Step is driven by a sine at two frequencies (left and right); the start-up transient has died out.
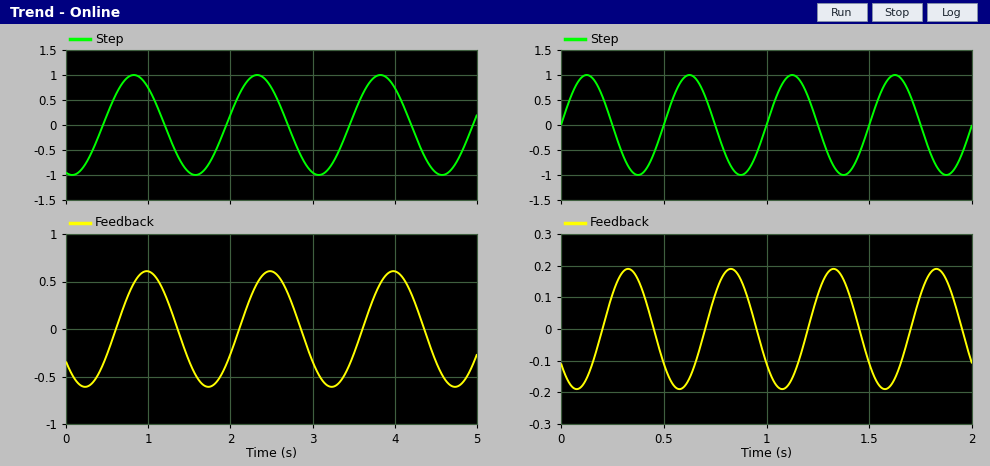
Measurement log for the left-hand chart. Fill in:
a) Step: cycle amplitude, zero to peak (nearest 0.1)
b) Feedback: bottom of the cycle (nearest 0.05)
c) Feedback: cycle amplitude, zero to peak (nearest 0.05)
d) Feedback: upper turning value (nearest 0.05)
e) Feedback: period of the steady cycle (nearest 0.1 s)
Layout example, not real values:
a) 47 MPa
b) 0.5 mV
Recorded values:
a) 1.0
b) -0.60
c) 0.60
d) 0.60
e) 1.5 s
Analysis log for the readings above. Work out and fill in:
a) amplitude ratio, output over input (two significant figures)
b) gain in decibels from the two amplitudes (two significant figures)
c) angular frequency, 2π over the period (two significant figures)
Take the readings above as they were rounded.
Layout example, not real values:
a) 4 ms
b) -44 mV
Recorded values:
a) 0.60
b) -4.4 dB
c) 4.2 rad/s
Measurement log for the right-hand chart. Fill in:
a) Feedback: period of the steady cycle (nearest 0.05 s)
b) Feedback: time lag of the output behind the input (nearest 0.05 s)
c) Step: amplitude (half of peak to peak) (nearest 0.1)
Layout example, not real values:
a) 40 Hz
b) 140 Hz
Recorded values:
a) 0.50 s
b) 0.20 s
c) 1.0
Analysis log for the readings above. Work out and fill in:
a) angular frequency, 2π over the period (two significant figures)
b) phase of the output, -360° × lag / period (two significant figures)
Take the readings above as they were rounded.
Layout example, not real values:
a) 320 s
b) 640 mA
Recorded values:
a) 13 rad/s
b) -140°
